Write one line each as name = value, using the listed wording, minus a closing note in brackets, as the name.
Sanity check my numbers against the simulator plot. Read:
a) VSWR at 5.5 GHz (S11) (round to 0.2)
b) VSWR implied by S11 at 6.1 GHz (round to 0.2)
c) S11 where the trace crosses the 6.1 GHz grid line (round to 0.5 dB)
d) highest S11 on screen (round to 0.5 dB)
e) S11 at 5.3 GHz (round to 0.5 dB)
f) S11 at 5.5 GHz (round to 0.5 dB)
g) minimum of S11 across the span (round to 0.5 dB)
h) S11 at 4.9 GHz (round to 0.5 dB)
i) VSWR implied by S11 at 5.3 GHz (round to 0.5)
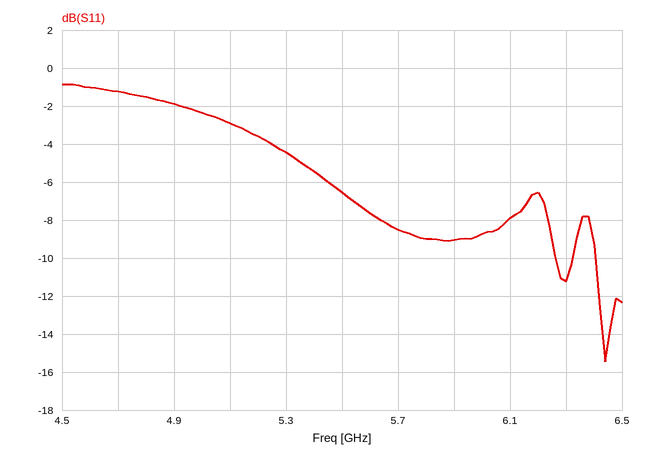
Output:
VSWR at 5.5 GHz (S11) = 2.8
VSWR implied by S11 at 6.1 GHz = 2.4
S11 where the trace crosses the 6.1 GHz grid line = -8.0 dB
highest S11 on screen = -1.0 dB
S11 at 5.3 GHz = -4.5 dB
S11 at 5.5 GHz = -6.5 dB
minimum of S11 across the span = -15.5 dB
S11 at 4.9 GHz = -2.0 dB
VSWR implied by S11 at 5.3 GHz = 4.0
